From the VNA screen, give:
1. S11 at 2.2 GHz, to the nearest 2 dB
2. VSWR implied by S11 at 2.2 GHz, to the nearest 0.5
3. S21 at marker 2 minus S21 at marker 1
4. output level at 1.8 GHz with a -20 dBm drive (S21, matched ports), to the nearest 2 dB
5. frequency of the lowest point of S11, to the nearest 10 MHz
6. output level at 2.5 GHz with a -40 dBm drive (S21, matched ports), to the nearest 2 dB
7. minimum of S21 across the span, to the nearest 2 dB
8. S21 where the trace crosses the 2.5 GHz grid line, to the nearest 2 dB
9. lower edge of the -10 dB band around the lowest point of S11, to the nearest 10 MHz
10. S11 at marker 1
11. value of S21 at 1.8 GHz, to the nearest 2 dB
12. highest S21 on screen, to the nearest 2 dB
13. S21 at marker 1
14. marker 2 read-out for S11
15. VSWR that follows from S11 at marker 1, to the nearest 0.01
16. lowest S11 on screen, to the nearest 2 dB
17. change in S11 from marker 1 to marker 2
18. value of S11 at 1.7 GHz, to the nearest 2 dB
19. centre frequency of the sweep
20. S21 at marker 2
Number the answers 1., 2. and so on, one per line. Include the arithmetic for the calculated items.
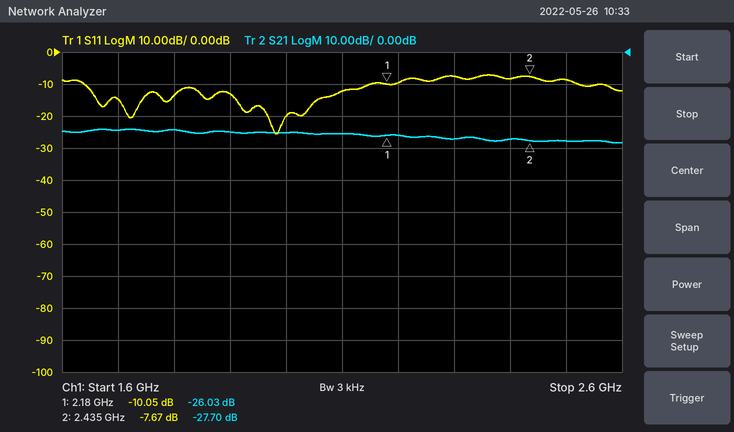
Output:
1. -10 dB
2. |Γ| = 10^(-10/20) = 0.3162; VSWR = (1 + 0.3162)/(1 − 0.3162) ≈ 1.92, so 2.0 to the nearest 0.5
3. -27.7 − (-26.03) = -1.67 dB
4. -20 dBm + (-24 dB) = -44 dBm
5. 1.98 GHz
6. -40 dBm + (-28 dB) = -68 dBm
7. -28 dB
8. -28 dB
9. 1.64 GHz
10. -10.05 dB
11. -24 dB
12. -24 dB
13. -26.03 dB
14. -7.67 dB
15. (1 + 0.3144)/(1 − 0.3144) ≈ 1.92
16. -26 dB
17. -7.67 − (-10.05) = 2.38 dB
18. -14 dB
19. 2.1 GHz
20. -27.70 dB
